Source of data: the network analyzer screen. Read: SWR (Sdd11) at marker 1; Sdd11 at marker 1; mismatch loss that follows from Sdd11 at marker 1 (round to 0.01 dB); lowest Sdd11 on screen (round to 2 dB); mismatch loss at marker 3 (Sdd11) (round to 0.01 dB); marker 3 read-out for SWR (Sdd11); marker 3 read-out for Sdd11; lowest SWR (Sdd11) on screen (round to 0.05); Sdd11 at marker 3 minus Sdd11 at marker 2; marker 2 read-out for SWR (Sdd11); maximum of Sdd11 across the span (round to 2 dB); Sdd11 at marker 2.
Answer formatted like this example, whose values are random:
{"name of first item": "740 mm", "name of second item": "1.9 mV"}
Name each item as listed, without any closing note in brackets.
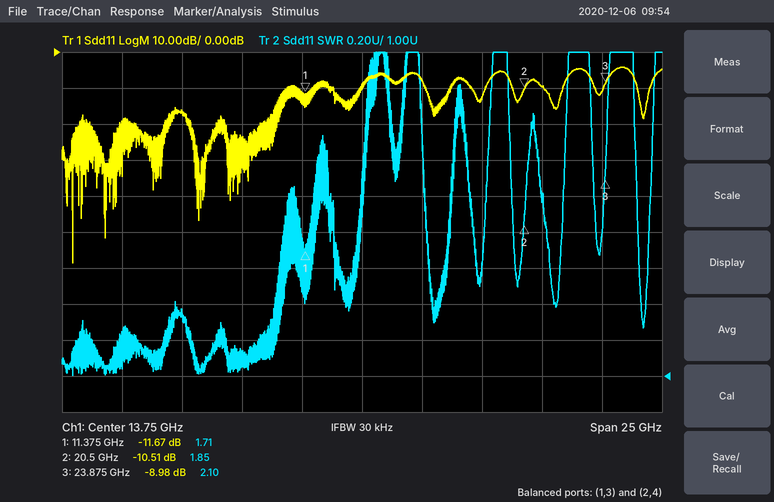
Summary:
{"SWR (Sdd11) at marker 1": "1.71", "Sdd11 at marker 1": "-11.67 dB", "mismatch loss that follows from Sdd11 at marker 1": "0.31 dB", "lowest Sdd11 on screen": "-58 dB", "mismatch loss at marker 3 (Sdd11)": "0.59 dB", "marker 3 read-out for SWR": "2.10", "marker 3 read-out for Sdd11": "-8.98 dB", "lowest SWR (Sdd11) on screen": "1.00", "Sdd11 at marker 3 minus Sdd11 at marker 2": "1.53 dB", "marker 2 read-out for SWR": "1.85", "maximum of Sdd11 across the span": "-4 dB", "Sdd11 at marker 2": "-10.51 dB"}
